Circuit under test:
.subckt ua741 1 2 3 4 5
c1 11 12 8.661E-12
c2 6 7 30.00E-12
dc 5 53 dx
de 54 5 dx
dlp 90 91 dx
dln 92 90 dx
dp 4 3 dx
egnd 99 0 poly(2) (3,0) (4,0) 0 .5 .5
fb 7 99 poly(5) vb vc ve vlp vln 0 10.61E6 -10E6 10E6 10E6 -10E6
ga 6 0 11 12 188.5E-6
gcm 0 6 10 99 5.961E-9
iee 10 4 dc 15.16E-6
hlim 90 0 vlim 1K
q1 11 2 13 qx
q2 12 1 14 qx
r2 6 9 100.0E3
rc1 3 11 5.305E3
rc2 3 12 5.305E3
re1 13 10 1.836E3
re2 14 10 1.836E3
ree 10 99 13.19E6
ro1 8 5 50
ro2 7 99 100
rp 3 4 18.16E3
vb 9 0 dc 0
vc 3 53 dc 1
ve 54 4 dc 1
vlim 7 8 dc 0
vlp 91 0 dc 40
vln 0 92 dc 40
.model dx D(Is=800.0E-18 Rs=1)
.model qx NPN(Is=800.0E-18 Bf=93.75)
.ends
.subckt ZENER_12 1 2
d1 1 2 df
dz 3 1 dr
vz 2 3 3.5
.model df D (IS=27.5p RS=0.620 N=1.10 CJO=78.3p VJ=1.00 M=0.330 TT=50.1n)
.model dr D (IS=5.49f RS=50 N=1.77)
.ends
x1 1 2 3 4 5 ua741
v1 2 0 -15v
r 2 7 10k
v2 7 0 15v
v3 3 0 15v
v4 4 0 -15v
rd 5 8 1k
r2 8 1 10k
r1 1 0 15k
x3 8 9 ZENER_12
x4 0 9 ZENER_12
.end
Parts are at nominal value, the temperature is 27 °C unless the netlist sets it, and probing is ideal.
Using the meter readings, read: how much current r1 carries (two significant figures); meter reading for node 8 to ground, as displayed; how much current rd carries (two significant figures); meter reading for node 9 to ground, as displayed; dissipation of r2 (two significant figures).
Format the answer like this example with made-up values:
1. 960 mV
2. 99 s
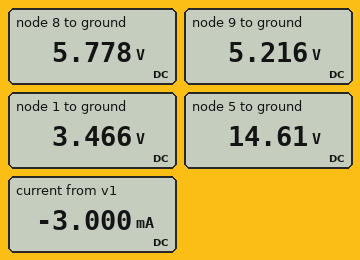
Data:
1. 230 µA
2. 5.778 V
3. 8.8 mA
4. 5.216 V
5. 530 µW
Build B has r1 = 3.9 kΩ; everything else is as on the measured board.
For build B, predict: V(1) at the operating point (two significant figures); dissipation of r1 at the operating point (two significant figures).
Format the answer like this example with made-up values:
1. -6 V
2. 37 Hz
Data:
1. 1.6 V
2. 670 µW
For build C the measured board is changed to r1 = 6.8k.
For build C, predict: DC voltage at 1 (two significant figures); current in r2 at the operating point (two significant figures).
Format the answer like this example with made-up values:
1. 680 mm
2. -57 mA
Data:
1. 2.3 V
2. 340 µA
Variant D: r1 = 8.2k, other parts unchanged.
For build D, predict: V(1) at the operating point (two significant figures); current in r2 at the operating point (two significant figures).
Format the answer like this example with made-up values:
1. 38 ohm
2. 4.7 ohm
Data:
1. 2.6 V
2. 320 µA
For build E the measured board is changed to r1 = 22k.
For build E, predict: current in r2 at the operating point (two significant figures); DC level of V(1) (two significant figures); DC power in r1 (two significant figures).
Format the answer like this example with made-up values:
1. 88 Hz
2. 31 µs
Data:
1. 180 µA
2. 4.0 V
3. 720 µW
